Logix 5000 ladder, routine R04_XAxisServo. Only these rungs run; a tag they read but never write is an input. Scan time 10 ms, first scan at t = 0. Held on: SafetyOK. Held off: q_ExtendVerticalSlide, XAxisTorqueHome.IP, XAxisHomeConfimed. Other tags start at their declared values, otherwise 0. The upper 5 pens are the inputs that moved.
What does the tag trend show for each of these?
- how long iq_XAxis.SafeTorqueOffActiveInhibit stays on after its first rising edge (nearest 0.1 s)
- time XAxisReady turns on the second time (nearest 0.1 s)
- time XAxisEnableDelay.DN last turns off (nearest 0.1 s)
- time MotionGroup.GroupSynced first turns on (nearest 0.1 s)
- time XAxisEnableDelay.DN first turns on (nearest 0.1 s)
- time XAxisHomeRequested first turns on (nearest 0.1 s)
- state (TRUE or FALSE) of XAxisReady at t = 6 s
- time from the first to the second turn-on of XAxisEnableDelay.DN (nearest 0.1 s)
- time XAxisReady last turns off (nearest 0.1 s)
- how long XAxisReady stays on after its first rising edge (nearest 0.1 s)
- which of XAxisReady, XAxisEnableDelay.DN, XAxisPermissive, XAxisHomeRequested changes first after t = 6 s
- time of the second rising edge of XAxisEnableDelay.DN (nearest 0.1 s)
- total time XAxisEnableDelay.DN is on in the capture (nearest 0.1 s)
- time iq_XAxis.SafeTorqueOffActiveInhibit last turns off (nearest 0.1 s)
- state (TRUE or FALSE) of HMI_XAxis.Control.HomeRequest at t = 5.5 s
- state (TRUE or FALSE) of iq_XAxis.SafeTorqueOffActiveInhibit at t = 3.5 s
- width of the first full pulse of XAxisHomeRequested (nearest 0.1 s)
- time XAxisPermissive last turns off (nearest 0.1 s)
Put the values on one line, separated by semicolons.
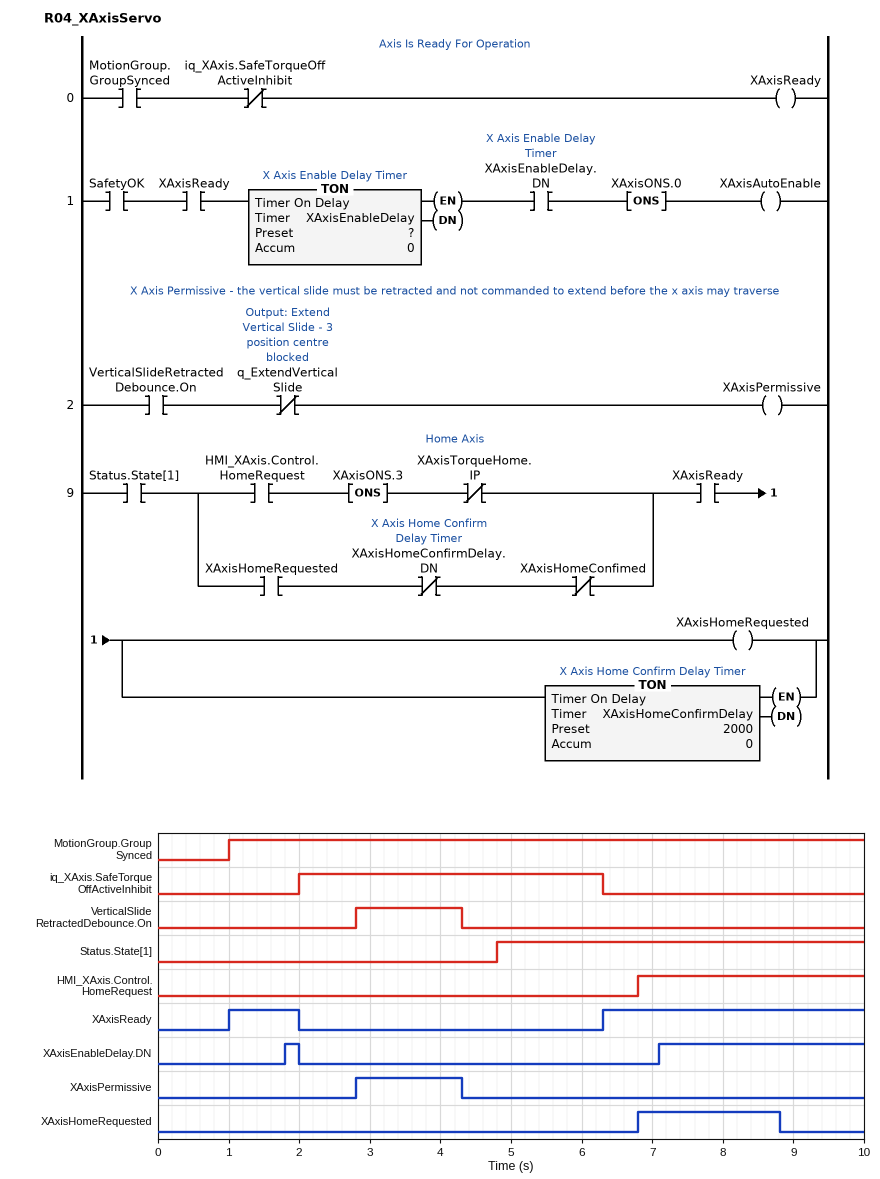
4.3 s; 6.3 s; 2.0 s; 1.0 s; 1.8 s; 6.8 s; FALSE; 5.3 s; 2.0 s; 1.0 s; XAxisReady; 7.1 s; 3.1 s; 6.3 s; FALSE; TRUE; 2.0 s; 4.3 s
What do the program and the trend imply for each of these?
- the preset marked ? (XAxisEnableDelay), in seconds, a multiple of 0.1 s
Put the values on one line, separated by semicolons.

0.8 s
